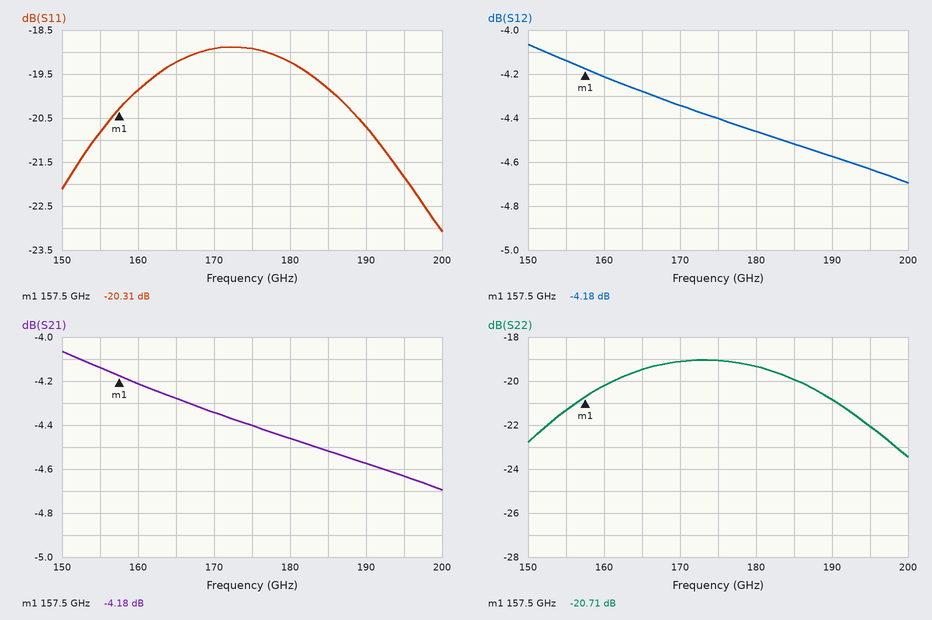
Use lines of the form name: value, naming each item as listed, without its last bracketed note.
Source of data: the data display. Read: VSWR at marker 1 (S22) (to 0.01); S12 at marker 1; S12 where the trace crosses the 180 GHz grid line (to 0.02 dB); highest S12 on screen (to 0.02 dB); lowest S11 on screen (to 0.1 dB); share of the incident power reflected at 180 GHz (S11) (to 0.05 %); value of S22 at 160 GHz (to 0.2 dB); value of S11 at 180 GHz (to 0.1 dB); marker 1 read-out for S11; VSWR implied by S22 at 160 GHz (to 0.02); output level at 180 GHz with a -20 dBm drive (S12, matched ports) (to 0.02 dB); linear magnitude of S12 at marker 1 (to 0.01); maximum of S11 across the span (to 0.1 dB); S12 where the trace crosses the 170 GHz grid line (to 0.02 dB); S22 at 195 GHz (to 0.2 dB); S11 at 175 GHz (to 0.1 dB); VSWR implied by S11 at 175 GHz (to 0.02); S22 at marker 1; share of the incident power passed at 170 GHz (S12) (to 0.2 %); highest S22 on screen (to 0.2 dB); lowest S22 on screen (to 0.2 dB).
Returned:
VSWR at marker 1 (S22): 1.20
S12 at marker 1: -4.18 dB
S12 where the trace crosses the 180 GHz grid line: -4.46 dB
highest S12 on screen: -4.06 dB
lowest S11 on screen: -23.1 dB
share of the incident power reflected at 180 GHz (S11): 1.20 %
value of S22 at 160 GHz: -20.2 dB
value of S11 at 180 GHz: -19.2 dB
marker 1 read-out for S11: -20.31 dB
VSWR implied by S22 at 160 GHz: 1.22
output level at 180 GHz with a -20 dBm drive (S12, matched ports): -24.46 dBm
linear magnitude of S12 at marker 1: 0.62
maximum of S11 across the span: -18.9 dB
S12 where the trace crosses the 170 GHz grid line: -4.34 dB
S22 at 195 GHz: -22.0 dB
S11 at 175 GHz: -18.9 dB
VSWR implied by S11 at 175 GHz: 1.26
S22 at marker 1: -20.71 dB
share of the incident power passed at 170 GHz (S12): 36.8 %
highest S22 on screen: -19.0 dB
lowest S22 on screen: -23.4 dB
